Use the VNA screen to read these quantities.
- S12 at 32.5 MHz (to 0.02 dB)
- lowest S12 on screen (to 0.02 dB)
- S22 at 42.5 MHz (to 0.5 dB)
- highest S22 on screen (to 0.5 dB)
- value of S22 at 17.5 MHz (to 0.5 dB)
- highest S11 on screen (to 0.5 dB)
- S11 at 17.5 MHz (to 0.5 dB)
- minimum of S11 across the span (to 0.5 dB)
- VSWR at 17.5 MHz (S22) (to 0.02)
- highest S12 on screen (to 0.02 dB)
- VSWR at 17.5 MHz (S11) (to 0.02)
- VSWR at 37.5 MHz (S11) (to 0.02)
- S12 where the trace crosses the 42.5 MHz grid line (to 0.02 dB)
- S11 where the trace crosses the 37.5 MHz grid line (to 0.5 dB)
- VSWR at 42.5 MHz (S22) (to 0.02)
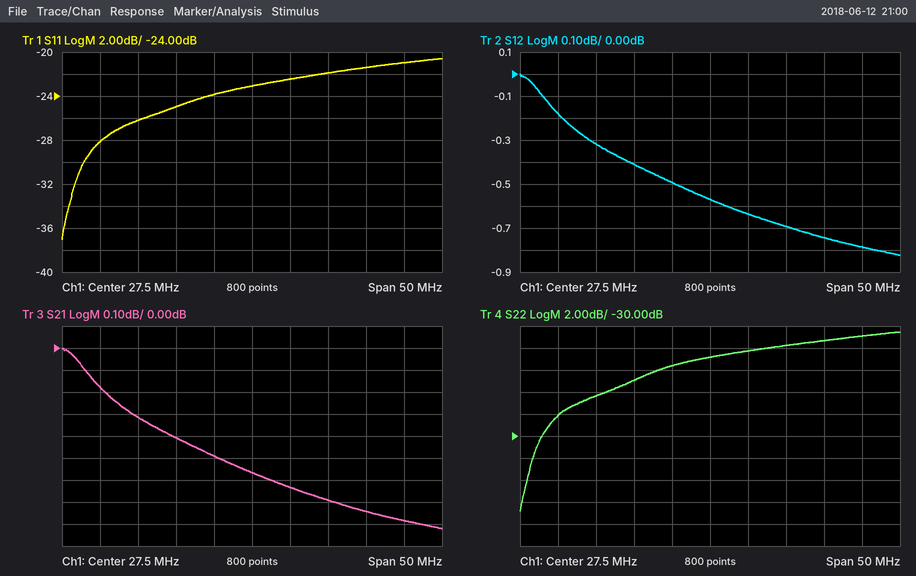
-0.64 dB
-0.82 dB
-21.5 dB
-20.5 dB
-25.0 dB
-20.5 dB
-25.0 dB
-37.0 dB
1.12
0.00 dB
1.12
1.18
-0.74 dB
-22.0 dB
1.18
